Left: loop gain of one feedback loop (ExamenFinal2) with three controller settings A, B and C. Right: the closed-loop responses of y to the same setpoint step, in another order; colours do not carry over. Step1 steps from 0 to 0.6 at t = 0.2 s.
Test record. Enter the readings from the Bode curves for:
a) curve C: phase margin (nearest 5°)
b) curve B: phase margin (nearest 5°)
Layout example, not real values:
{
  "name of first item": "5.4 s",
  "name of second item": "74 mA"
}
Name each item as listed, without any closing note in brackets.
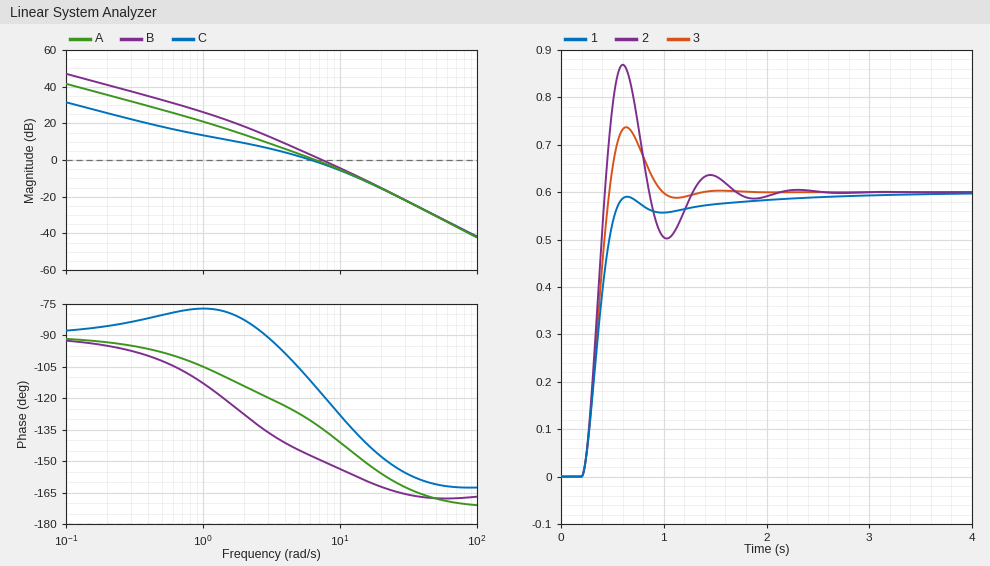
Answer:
{
  "curve C: phase margin": "70°",
  "curve B: phase margin": "30°"
}
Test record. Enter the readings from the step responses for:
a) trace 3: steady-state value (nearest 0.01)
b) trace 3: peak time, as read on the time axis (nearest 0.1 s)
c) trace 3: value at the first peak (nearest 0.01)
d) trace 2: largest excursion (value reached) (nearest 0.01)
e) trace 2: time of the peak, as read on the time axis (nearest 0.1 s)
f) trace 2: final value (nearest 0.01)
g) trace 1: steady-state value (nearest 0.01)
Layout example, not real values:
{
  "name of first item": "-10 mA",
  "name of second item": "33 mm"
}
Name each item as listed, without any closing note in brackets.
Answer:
{
  "trace 3: steady-state value": "0.60",
  "trace 3: peak time, as read on the time axis": "0.6 s",
  "trace 3: value at the first peak": "0.74",
  "trace 2: largest excursion (value reached)": "0.87",
  "trace 2: time of the peak, as read on the time axis": "0.6 s",
  "trace 2: final value": "0.60",
  "trace 1: steady-state value": "0.60"
}
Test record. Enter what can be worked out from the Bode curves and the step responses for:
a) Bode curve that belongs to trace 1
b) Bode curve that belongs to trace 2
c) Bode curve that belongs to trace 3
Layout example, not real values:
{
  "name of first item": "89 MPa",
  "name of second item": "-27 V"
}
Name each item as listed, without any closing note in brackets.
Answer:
{
  "Bode curve that belongs to trace 1": "C",
  "Bode curve that belongs to trace 2": "B",
  "Bode curve that belongs to trace 3": "A"
}
